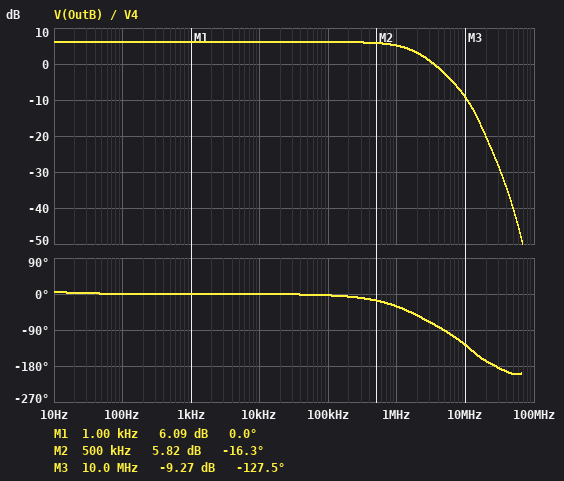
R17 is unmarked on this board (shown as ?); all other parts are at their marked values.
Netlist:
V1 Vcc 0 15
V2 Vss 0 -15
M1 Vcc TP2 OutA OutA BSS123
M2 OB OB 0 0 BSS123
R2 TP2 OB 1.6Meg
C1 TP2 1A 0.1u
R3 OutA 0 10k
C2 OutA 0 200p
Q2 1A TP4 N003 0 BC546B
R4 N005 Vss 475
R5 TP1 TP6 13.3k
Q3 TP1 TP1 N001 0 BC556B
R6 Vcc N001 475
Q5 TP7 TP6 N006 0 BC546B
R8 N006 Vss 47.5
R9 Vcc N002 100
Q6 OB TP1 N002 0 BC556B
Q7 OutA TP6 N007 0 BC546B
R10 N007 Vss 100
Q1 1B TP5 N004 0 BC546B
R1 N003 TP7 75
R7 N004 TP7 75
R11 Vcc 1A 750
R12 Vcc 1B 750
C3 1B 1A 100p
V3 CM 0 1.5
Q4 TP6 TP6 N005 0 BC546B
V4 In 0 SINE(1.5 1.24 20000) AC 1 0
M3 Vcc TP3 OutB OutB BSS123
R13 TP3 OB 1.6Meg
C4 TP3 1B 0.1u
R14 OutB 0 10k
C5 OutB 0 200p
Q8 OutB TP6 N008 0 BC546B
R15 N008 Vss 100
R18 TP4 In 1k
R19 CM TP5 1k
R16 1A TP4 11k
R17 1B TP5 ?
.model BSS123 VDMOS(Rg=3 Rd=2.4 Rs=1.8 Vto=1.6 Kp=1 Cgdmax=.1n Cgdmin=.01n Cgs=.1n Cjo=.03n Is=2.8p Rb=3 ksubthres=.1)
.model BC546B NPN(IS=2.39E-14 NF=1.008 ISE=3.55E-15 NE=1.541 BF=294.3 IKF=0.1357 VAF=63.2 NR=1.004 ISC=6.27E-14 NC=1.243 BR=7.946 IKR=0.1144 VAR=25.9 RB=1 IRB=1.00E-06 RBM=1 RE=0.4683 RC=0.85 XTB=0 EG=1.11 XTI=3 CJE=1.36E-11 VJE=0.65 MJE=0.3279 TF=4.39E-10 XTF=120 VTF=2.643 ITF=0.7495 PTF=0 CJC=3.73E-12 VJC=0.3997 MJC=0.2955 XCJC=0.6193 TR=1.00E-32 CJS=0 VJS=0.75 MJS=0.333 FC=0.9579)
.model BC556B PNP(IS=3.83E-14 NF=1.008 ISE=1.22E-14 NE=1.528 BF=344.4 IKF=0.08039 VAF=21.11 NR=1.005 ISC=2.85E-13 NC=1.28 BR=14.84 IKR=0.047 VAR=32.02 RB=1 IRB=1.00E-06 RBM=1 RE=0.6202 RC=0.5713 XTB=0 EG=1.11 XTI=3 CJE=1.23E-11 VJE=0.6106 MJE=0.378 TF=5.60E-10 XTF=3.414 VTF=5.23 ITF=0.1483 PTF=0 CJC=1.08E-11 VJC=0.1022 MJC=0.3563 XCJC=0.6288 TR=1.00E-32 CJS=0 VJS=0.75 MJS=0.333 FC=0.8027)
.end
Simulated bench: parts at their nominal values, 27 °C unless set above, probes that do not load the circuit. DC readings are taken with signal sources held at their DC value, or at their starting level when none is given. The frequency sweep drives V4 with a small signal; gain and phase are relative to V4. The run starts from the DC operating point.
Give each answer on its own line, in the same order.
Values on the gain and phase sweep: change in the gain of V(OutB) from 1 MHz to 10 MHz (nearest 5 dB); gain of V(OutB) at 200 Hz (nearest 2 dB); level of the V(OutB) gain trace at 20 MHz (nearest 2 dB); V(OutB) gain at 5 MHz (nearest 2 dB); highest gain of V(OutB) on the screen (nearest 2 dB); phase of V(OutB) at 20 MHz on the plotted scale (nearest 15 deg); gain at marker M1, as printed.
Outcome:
-15 dB
6 dB
-20 dB
-2 dB
6 dB
-165 deg
6.09 dB
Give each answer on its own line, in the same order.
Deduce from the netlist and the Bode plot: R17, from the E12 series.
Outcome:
6.8 kΩ
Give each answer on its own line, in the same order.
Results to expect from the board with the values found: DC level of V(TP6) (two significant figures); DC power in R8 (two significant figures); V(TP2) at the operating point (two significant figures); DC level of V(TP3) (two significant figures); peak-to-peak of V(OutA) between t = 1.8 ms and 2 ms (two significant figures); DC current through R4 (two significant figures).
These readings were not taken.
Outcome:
-13 V
15 mW
1.7 V
1.7 V
5.0 V
1.9 mA
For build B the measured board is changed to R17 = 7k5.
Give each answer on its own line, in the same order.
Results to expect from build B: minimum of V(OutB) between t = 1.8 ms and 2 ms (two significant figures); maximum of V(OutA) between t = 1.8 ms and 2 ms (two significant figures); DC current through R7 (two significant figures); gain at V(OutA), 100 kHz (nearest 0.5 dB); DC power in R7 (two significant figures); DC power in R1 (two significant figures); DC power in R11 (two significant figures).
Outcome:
-2.6 V
2.6 V
9.5 mA
6.5 dB
6.8 mW
5.0 mW
57 mW
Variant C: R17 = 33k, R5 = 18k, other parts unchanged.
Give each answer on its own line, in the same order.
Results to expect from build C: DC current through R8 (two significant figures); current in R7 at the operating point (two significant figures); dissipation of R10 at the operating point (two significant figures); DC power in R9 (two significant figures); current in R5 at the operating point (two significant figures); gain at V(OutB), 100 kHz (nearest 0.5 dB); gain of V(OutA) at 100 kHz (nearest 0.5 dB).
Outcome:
13 mA
4.8 mA
4.2 mW
4.7 mW
1.5 mA
8.5 dB
8.0 dB
